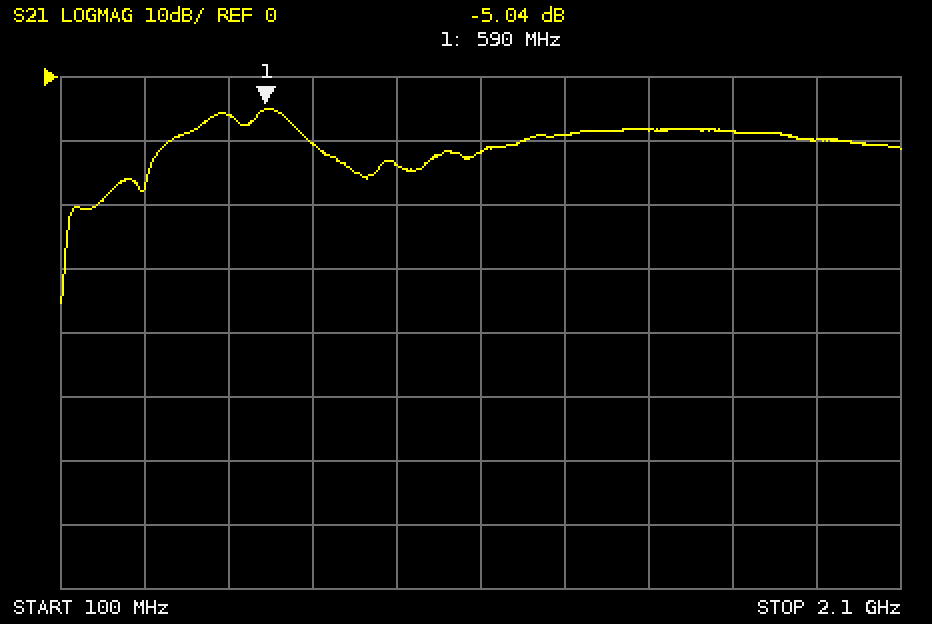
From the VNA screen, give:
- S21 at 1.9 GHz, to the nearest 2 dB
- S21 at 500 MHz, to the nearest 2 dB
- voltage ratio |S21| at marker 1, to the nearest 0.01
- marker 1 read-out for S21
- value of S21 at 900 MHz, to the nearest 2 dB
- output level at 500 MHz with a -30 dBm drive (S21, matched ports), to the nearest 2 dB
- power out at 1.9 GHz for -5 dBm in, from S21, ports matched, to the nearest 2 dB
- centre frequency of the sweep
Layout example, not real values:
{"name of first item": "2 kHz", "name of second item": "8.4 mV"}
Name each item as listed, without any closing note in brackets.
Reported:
{"S21 at 1.9 GHz, to the nearest 2 dB": "-10 dB", "S21 at 500 MHz, to the nearest 2 dB": "-6 dB", "voltage ratio |S21| at marker 1, to the nearest 0.01": "0.56", "marker 1 read-out for S21": "-5.04 dB", "value of S21 at 900 MHz, to the nearest 2 dB": "-14 dB", "output level at 500 MHz with a -30 dBm drive (S21, matched ports), to the nearest 2 dB": "-36 dBm", "power out at 1.9 GHz for -5 dBm in, from S21, ports matched, to the nearest 2 dB": "-14 dBm", "centre frequency of the sweep": "1.1 GHz"}
